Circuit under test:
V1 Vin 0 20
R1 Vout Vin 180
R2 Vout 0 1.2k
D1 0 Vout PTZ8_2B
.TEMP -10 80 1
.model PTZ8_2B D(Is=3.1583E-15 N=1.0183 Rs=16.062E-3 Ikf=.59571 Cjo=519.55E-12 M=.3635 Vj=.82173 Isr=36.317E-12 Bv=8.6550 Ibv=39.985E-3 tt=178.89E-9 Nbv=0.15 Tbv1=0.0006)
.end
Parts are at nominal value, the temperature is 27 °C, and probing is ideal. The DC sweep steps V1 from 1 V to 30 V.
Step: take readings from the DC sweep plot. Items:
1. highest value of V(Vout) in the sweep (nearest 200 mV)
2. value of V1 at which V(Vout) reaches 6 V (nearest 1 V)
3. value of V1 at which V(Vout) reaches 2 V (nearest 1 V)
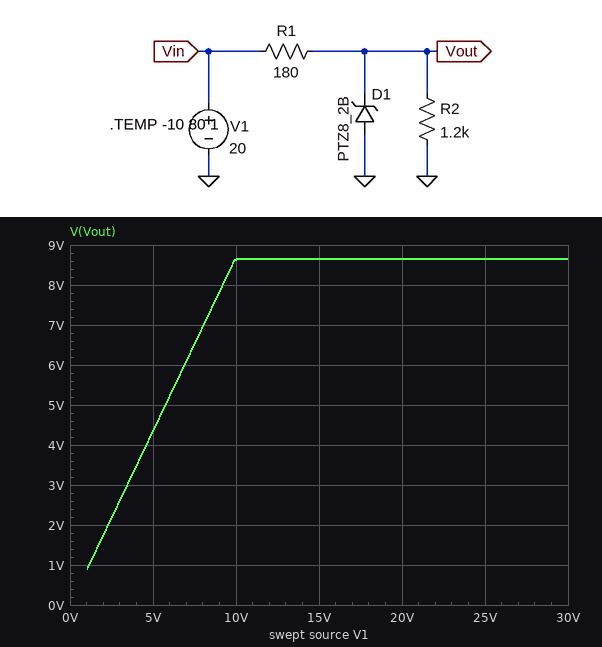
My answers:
8.6 V
7 V
2 V
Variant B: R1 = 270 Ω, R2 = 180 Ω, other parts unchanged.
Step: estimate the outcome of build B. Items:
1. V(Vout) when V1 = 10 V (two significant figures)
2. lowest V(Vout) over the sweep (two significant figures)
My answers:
4.0 V
400 mV
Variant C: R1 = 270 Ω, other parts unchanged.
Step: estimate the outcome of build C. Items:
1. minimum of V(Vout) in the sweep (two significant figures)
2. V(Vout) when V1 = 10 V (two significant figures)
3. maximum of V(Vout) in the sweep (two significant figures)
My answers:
820 mV
8.2 V
8.7 V
